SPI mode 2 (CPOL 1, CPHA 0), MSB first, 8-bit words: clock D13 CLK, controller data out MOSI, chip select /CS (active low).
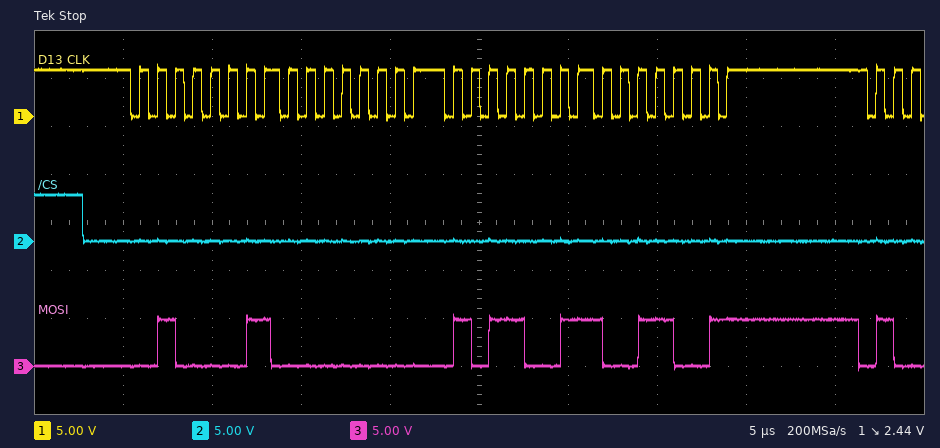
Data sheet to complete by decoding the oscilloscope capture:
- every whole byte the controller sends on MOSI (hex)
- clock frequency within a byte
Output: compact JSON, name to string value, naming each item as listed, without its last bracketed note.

{"every whole byte the controller sends on MOSI": "0x21 0x00 0x59 0x99", "clock frequency within a byte": "1 MHz"}
